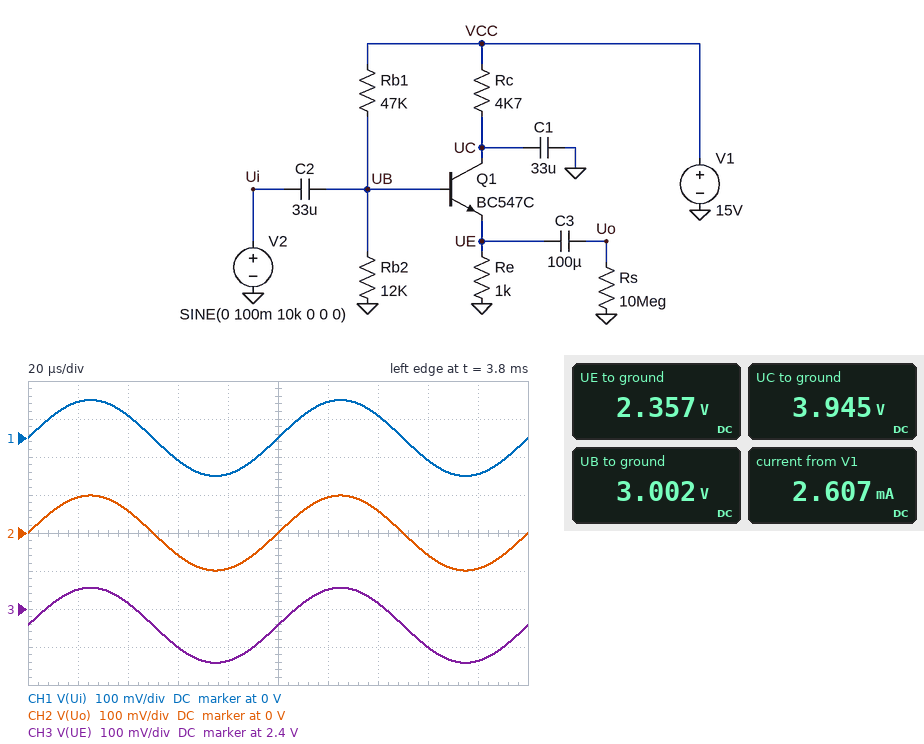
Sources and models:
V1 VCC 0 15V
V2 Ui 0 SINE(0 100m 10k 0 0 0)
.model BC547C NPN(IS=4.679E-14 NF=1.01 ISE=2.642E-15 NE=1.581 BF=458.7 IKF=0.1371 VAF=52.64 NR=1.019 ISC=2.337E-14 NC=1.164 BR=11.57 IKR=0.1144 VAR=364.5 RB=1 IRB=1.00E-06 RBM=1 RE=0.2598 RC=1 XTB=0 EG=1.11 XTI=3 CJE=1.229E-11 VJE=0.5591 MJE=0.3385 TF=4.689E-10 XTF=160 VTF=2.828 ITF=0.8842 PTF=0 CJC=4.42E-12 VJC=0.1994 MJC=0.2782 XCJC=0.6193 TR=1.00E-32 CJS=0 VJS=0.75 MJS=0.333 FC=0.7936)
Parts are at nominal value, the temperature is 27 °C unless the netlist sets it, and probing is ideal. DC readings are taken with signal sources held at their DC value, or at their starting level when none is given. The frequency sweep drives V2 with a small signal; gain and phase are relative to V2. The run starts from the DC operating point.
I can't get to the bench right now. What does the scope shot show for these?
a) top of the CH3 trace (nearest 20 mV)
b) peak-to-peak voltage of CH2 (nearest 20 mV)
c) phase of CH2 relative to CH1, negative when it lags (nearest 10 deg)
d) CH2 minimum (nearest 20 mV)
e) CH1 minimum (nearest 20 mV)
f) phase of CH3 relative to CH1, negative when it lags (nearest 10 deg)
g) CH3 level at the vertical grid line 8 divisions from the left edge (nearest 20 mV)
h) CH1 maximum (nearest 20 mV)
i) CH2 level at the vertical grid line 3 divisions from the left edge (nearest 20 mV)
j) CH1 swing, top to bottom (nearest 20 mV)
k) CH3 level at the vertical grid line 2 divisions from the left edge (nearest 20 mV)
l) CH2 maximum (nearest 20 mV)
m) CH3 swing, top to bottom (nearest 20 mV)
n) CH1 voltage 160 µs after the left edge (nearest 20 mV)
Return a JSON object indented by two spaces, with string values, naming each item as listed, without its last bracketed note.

{
  "top of the CH3 trace": "2.46 V",
  "peak-to-peak voltage of CH2": "200 mV",
  "phase of CH2 relative to CH1, negative when it lags": "0 deg",
  "CH2 minimum": "-100 mV",
  "CH1 minimum": "-100 mV",
  "phase of CH3 relative to CH1, negative when it lags": "0 deg",
  "CH3 level at the vertical grid line 8 divisions from the left edge": "2.30 V",
  "CH1 maximum": "100 mV",
  "CH2 level at the vertical grid line 3 divisions from the left edge": "-60 mV",
  "CH1 swing, top to bottom": "200 mV",
  "CH3 level at the vertical grid line 2 divisions from the left edge": "2.42 V",
  "CH2 maximum": "100 mV",
  "CH3 swing, top to bottom": "200 mV",
  "CH1 voltage 160 µs after the left edge": "-60 mV"
}
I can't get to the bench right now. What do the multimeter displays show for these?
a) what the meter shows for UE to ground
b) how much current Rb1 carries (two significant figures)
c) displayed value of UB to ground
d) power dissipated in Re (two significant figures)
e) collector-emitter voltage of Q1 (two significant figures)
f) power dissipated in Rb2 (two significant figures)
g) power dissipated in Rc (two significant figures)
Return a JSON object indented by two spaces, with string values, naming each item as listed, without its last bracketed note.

{
  "what the meter shows for UE to ground": "2.357 V",
  "how much current Rb1 carries": "260 µA",
  "displayed value of UB to ground": "3.002 V",
  "power dissipated in Re": "5.6 mW",
  "collector-emitter voltage of Q1": "1.6 V",
  "power dissipated in Rb2": "750 µW",
  "power dissipated in Rc": "26 mW"
}
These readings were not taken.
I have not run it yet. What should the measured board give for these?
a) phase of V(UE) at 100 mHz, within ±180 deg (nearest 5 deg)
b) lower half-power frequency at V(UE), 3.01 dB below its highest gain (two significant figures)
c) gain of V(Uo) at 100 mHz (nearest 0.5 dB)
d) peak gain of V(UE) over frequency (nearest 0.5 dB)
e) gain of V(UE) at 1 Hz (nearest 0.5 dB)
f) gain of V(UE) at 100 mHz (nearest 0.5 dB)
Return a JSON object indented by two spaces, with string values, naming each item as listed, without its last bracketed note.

{
  "phase of V(UE) at 100 mHz, within ±180 deg": "80 deg",
  "lower half-power frequency at V(UE), 3.01 dB below its highest gain": "520 mHz",
  "gain of V(Uo) at 100 mHz": "-14.5 dB",
  "peak gain of V(UE) over frequency": "0 dB",
  "gain of V(UE) at 1 Hz": "-1.0 dB",
  "gain of V(UE) at 100 mHz": "-14.5 dB"
}
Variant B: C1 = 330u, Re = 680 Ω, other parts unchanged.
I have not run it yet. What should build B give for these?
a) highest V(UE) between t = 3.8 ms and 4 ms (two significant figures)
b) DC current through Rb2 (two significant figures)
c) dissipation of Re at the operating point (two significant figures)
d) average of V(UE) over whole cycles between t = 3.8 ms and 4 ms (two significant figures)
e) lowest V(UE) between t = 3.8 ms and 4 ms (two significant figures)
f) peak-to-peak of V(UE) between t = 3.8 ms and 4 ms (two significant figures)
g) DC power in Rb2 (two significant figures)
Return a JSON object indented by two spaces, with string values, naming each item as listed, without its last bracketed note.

{
  "highest V(UE) between t = 3.8 ms and 4 ms": "2.0 V",
  "DC current through Rb2": "210 µA",
  "dissipation of Re at the operating point": "5.4 mW",
  "average of V(UE) over whole cycles between t = 3.8 ms and 4 ms": "1.9 V",
  "lowest V(UE) between t = 3.8 ms and 4 ms": "1.8 V",
  "peak-to-peak of V(UE) between t = 3.8 ms and 4 ms": "170 mV",
  "DC power in Rb2": "550 µW"
}
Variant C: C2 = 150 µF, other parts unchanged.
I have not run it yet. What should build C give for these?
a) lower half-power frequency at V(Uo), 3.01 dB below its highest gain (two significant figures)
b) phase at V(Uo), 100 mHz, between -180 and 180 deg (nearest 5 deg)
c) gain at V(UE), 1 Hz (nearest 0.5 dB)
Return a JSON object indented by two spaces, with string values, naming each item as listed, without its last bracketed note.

{
  "lower half-power frequency at V(Uo), 3.01 dB below its highest gain": "110 mHz",
  "phase at V(Uo), 100 mHz, between -180 and 180 deg": "50 deg",
  "gain at V(UE), 1 Hz": "0 dB"
}
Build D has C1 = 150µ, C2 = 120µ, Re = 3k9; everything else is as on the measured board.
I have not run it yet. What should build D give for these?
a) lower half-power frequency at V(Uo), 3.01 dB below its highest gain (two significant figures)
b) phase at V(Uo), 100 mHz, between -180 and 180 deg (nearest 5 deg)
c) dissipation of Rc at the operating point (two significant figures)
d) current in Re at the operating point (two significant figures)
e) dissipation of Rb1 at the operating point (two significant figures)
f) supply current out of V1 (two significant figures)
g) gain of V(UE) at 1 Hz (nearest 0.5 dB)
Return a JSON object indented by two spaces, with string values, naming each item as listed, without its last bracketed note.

{
  "lower half-power frequency at V(Uo), 3.01 dB below its highest gain": "140 mHz",
  "phase at V(Uo), 100 mHz, between -180 and 180 deg": "55 deg",
  "dissipation of Rc at the operating point": "1.8 mW",
  "current in Re at the operating point": "620 µA",
  "dissipation of Rb1 at the operating point": "3.0 mW",
  "supply current out of V1": "880 µA",
  "gain of V(UE) at 1 Hz": "0 dB"
}
